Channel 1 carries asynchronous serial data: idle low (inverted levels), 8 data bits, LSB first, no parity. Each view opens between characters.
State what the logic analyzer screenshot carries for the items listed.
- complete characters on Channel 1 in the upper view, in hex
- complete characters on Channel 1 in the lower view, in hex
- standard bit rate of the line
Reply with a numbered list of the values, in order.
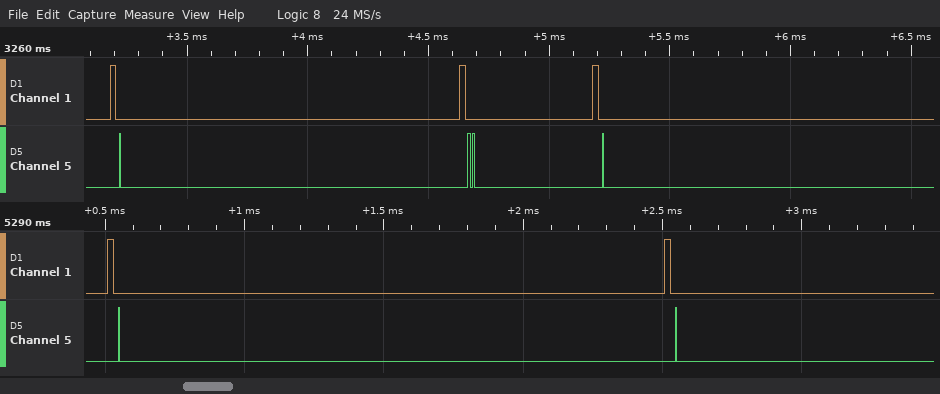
1. FF, FF, FF
2. FF, FF
3. 38400 baud
